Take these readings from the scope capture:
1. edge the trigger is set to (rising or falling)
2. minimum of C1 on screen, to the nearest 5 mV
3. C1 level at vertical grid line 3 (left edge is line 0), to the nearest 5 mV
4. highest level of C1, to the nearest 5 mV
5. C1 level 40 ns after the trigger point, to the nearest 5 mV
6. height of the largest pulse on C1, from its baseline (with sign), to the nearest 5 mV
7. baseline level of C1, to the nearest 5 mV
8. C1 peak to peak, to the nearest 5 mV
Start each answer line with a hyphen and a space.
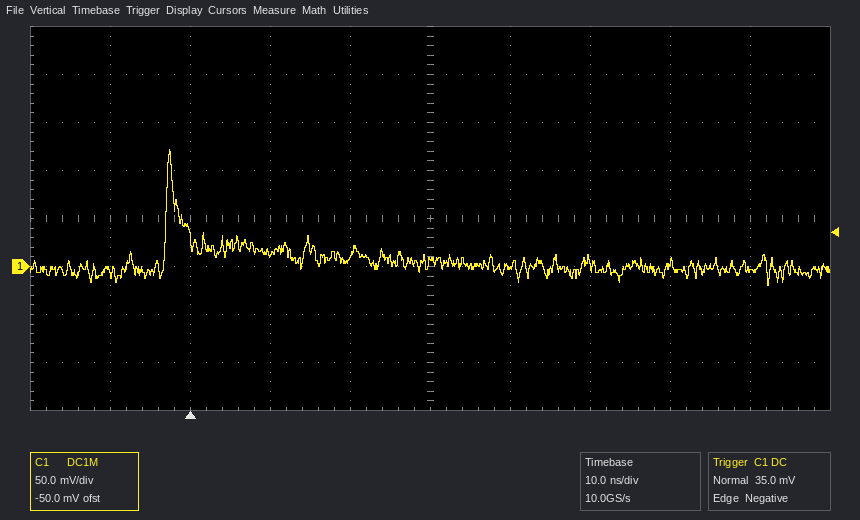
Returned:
- falling
- -20 mV
- 15 mV
- 120 mV
- 0 mV
- +120 mV
- 0 mV
- 140 mV
